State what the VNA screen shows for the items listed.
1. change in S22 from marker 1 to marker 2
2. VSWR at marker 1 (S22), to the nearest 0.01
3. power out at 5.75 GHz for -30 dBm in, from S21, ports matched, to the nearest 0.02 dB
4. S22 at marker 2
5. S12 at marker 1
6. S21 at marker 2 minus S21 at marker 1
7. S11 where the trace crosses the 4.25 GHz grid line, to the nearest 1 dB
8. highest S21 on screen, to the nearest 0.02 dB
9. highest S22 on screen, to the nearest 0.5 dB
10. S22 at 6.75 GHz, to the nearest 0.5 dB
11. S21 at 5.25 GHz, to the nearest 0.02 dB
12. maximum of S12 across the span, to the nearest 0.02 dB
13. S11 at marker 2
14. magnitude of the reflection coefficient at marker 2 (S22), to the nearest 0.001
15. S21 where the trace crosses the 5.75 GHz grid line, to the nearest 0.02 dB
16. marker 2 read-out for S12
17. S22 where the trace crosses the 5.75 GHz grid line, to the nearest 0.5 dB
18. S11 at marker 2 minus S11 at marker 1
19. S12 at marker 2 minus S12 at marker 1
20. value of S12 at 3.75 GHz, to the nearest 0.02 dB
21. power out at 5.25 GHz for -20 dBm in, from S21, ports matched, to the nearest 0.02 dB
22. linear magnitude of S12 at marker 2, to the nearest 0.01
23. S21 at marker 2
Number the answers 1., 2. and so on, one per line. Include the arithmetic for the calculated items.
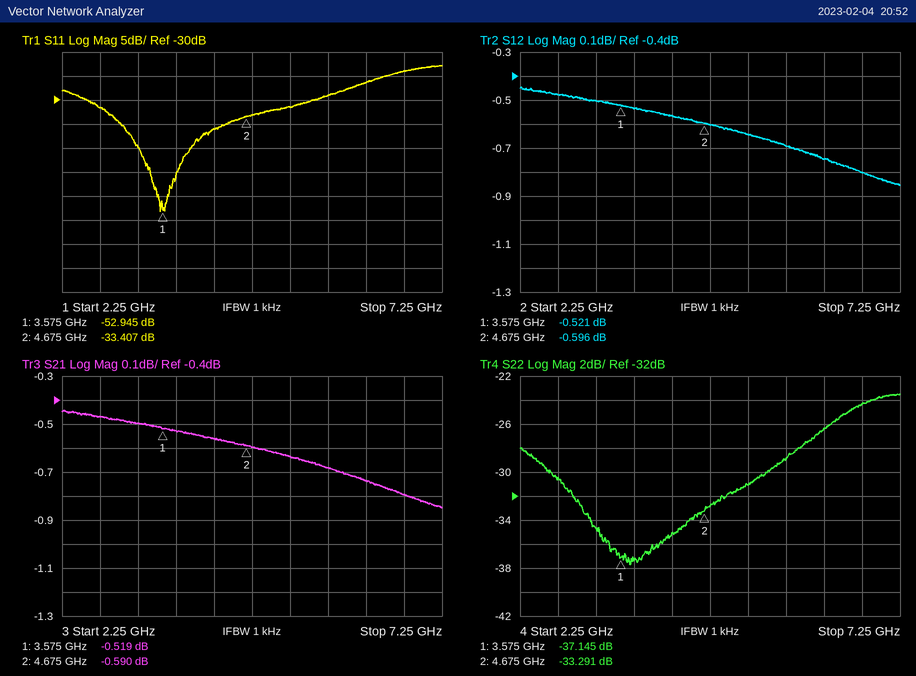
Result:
1. -33.291 − (-37.145) = 3.854 dB
2. (1 + 0.0139)/(1 − 0.0139) ≈ 1.03
3. -30 dBm + (-0.68 dB) = -30.68 dBm
4. -33.291 dB
5. -0.521 dB
6. -0.59 − (-0.519) = -0.071 dB
7. -36 dB
8. -0.44 dB
9. -23.5 dB
10. -24.5 dB
11. -0.64 dB
12. -0.44 dB
13. -33.407 dB
14. 10^(-33.291/20) ≈ 0.022
15. -0.68 dB
16. -0.596 dB
17. -29.0 dB
18. -33.407 − (-52.945) = 19.538 dB
19. -0.596 − (-0.521) = -0.075 dB
20. -0.54 dB
21. -20 dBm + (-0.64 dB) = -20.64 dBm
22. 10^(-0.596/20) ≈ 0.93
23. -0.590 dB
